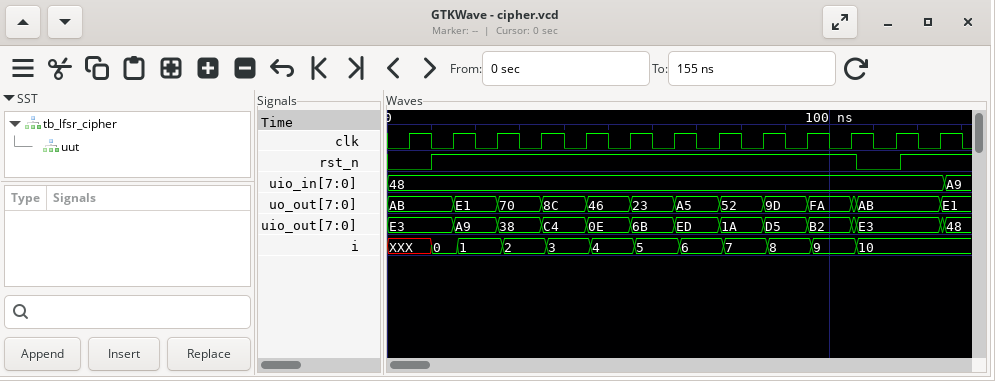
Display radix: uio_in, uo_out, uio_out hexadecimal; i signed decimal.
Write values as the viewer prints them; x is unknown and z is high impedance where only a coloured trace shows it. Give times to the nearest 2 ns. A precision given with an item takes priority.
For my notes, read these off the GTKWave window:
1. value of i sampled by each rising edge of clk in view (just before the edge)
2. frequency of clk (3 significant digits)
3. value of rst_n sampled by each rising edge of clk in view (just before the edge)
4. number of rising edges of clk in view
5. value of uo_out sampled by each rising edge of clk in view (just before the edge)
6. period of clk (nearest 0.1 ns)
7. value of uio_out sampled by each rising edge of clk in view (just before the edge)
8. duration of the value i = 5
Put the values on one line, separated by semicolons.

XXX, 0, 1, 2, 3, 4, 5, 6, 7, 8, 9, 10, 10; 100 MHz; 0 1 1 1 1 1 1 1 1 1 1 0 1; 13; AB, AB, E1, 70, 8C, 46, 23, A5, 52, 9D, FA, AB, AB; 10 ns; E3, E3, A9, 38, C4, 0E, 6B, ED, 1A, D5, B2, E3, E3; 10 ns
